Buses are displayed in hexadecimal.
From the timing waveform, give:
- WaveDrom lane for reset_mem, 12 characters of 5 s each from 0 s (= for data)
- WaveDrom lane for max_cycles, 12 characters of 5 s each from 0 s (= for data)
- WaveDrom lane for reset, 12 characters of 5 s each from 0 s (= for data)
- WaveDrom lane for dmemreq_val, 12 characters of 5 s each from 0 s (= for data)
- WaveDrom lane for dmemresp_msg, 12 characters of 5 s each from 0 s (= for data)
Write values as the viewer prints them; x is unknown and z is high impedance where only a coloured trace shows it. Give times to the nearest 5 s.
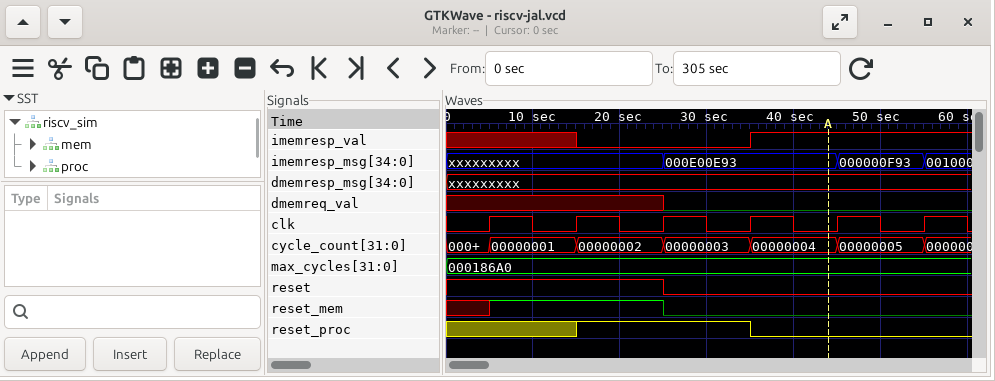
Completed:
{name: 'reset_mem', wave: 'x1...0......'}
{name: 'max_cycles', wave: '=...........', data: '000186A0'}
{name: 'reset', wave: '1....0......'}
{name: 'dmemreq_val', wave: 'x....0......'}
{name: 'dmemresp_msg', wave: 'x...........'}
